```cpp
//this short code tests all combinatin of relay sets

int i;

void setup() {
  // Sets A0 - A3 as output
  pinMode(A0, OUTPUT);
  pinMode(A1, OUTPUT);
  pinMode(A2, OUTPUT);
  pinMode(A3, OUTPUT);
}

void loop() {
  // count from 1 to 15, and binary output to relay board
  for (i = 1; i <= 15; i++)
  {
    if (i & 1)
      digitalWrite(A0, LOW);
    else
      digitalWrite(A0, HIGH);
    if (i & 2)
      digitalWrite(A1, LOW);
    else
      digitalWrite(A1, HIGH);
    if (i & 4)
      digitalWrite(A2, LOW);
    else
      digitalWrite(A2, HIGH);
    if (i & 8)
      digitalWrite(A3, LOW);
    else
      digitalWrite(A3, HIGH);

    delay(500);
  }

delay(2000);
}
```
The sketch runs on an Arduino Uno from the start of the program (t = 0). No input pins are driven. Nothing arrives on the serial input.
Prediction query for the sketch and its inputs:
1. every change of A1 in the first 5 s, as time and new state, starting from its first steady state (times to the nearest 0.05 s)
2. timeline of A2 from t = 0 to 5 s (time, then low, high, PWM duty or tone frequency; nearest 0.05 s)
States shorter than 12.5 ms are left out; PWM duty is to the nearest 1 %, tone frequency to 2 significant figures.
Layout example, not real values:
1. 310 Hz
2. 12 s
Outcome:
1. 0 s high; 0.5 s low; 1.5 s high; 2.5 s low; 3.5 s high; 4.5 s low
2. 0 s high; 1.5 s low; 3.5 s high
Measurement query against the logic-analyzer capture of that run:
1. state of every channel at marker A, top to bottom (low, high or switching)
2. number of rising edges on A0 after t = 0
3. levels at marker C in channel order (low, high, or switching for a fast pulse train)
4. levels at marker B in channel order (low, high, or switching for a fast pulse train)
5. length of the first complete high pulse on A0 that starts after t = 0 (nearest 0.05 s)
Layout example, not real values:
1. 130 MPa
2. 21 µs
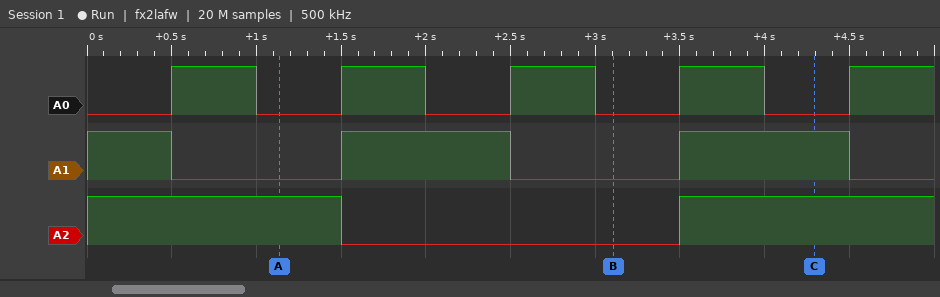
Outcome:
1. A0 low, A1 low, A2 high
2. 5
3. A0 low, A1 high, A2 high
4. A0 low, A1 low, A2 low
5. 0.50 s
